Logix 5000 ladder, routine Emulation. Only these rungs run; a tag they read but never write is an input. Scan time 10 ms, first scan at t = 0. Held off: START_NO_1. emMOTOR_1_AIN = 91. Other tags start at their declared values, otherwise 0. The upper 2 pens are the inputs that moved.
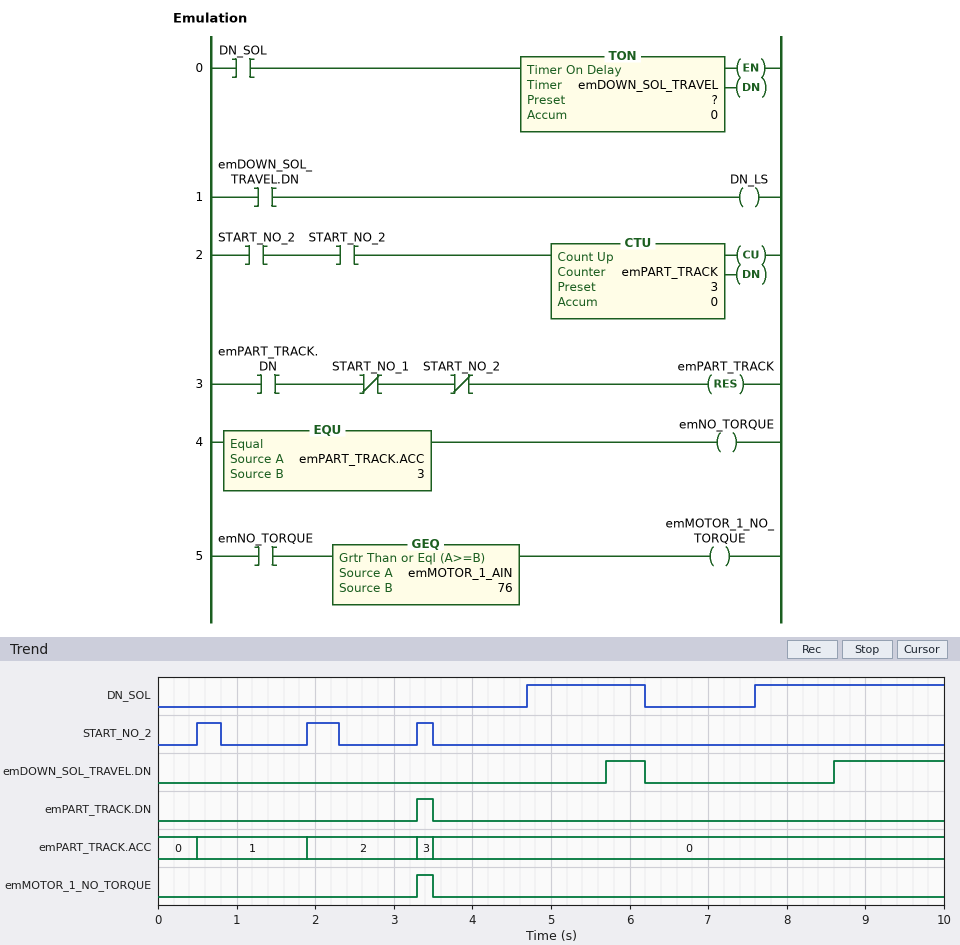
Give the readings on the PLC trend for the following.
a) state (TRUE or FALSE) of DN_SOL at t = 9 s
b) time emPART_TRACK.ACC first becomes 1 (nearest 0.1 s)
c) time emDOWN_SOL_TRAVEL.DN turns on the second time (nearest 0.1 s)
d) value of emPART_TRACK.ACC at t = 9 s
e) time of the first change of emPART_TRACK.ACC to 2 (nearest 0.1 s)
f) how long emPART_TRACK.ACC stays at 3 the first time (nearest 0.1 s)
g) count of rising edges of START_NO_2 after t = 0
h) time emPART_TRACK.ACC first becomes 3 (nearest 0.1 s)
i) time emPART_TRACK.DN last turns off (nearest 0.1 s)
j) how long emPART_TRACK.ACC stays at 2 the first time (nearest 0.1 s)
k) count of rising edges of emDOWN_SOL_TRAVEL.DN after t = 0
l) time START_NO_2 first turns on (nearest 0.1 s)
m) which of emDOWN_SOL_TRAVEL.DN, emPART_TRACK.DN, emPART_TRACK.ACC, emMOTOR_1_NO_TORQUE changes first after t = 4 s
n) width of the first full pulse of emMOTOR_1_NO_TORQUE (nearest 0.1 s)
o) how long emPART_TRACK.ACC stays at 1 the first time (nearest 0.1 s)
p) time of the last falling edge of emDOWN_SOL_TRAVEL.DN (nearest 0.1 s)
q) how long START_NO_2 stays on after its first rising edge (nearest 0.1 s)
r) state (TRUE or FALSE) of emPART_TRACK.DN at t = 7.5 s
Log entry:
TRUE
0.5 s
8.6 s
0
1.9 s
0.2 s
3
3.3 s
3.5 s
1.4 s
2
0.5 s
emDOWN_SOL_TRAVEL.DN
0.2 s
1.4 s
6.2 s
0.3 s
FALSE
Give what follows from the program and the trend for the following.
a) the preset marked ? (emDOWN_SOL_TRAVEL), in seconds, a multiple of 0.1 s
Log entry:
1.0 s
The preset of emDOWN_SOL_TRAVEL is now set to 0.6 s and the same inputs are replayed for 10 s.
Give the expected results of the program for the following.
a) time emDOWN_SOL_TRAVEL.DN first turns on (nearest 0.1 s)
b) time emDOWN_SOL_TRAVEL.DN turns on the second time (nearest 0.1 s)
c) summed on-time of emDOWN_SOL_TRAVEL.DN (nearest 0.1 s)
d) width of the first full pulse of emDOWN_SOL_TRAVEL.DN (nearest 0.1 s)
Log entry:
5.3 s
8.2 s
2.7 s
0.9 s
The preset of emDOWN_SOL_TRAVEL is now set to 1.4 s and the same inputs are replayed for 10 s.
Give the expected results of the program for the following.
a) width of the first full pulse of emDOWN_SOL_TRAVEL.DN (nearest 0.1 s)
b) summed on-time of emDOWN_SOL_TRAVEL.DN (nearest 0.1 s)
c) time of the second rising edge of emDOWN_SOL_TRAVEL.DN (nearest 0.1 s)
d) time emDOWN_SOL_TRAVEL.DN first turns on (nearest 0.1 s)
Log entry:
0.1 s
1.1 s
9.0 s
6.1 s
